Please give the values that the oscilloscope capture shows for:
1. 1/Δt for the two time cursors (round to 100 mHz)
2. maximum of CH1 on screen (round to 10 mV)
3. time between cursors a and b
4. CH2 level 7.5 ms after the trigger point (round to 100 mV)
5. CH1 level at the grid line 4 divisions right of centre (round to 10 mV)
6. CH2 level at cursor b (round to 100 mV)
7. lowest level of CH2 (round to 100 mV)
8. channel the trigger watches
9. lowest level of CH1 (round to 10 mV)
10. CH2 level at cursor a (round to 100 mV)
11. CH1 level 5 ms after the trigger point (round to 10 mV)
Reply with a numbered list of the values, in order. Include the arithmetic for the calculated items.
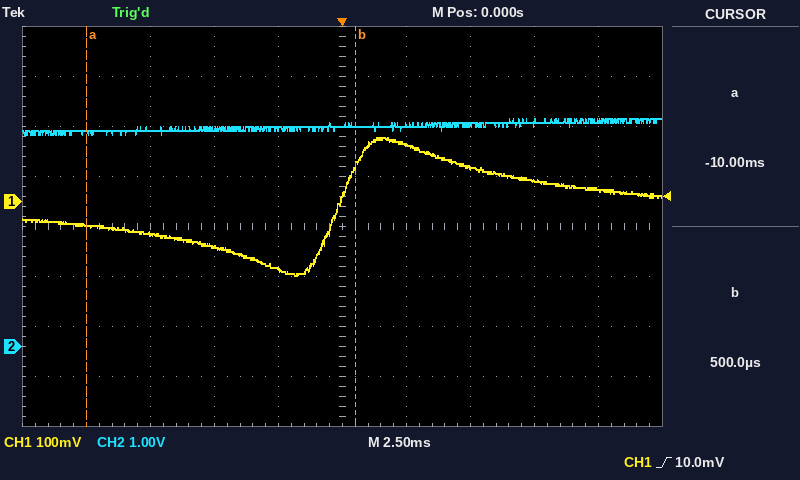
1. 1 / 10.50 ms ≈ 95.2 Hz
2. 130 mV
3. 500 µs − (-10 ms) = 10.50 ms
4. 4.5 V
5. 20 mV
6. 4.4 V
7. 4.2 V
8. CH1
9. -150 mV
10. 4.3 V
11. 70 mV
